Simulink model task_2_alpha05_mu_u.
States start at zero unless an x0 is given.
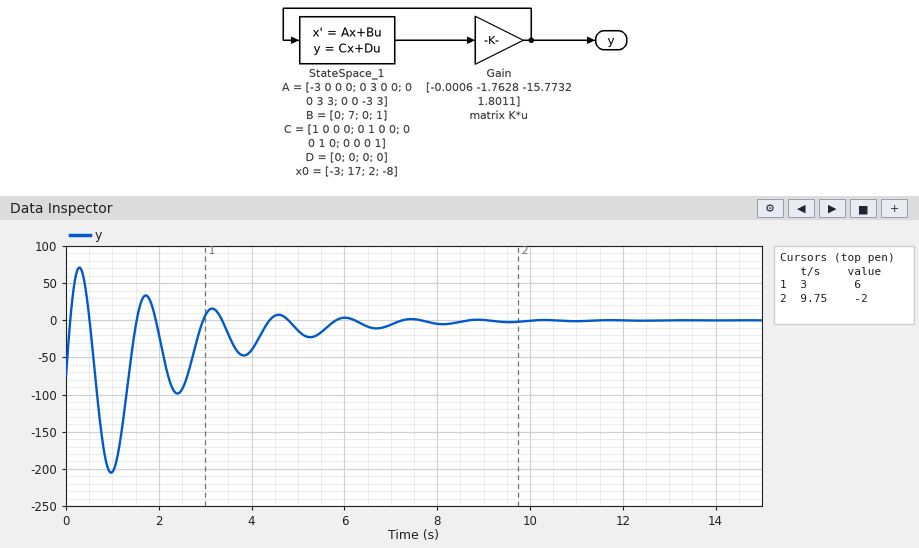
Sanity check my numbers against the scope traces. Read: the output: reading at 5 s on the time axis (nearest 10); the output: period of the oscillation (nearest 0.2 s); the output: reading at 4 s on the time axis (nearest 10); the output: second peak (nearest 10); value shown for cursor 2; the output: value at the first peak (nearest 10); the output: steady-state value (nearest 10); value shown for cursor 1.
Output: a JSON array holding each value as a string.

["-10", "1.4 s", "-40", "30", "-2", "70", "0", "6"]
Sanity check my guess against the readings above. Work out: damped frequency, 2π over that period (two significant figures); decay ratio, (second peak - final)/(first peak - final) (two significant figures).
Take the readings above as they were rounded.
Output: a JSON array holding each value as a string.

["4.5 rad/s", "0.43"]
